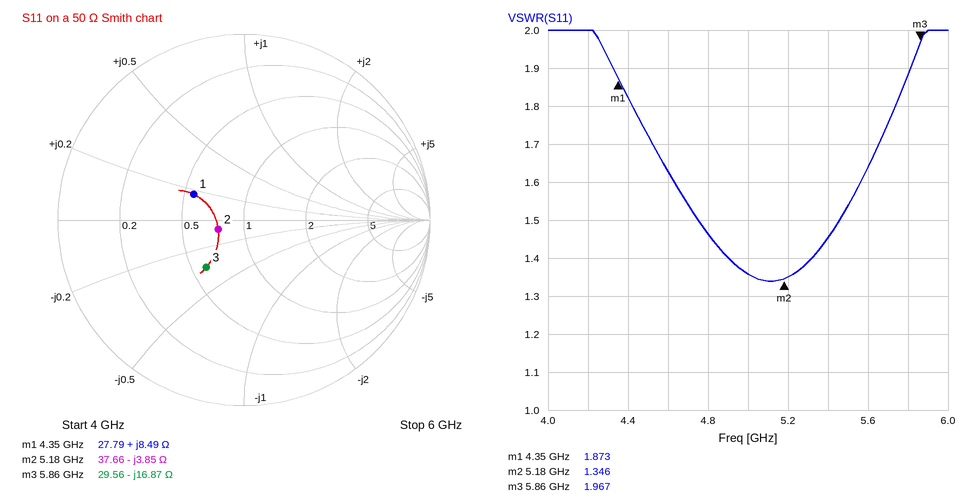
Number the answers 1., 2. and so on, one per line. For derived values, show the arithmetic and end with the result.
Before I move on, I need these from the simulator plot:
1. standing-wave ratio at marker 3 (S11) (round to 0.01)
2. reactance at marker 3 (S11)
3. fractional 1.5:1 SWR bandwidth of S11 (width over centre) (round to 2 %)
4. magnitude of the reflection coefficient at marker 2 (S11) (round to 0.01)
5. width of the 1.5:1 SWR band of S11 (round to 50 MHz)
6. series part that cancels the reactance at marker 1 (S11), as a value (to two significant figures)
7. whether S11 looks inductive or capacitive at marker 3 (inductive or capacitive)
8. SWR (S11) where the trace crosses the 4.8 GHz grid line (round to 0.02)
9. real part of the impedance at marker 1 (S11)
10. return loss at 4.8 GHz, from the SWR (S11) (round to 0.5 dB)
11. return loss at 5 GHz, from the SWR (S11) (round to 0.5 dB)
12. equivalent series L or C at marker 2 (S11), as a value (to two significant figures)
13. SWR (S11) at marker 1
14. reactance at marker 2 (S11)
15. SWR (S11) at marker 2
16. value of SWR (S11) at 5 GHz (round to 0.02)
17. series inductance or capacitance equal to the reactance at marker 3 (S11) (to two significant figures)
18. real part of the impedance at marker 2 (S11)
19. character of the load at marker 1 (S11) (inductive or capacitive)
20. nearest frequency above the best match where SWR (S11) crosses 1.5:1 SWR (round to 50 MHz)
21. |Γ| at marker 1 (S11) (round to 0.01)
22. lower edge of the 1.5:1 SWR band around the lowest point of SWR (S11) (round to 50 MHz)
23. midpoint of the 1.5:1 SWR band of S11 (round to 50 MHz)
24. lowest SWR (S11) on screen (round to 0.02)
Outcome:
1. 1.97
2. -16.87 Ω
3. 700 MHz / 5.1 GHz ≈ 14 %
4. 0.15
5. 5.45 GHz − 4.75 GHz = 700 MHz
6. C = 1/(2π × 4.35 GHz × 8.49 Ω) ≈ 4.3 pF
7. capacitive
8. 1.46
9. 27.79 Ω
10. −20 log10((1.46 − 1)/(1.46 + 1)) ≈ 14.6 dB, so 14.5 dB to the nearest 0.5 dB
11. −20 log10((1.36 − 1)/(1.36 + 1)) ≈ 16.3 dB, so 16.5 dB to the nearest 0.5 dB
12. C = 1/(2π × 5.18 GHz × 3.85 Ω) ≈ 8.0 pF
13. 1.873
14. -3.85 Ω
15. 1.346
16. 1.36
17. C = 1/(2π × 5.86 GHz × 16.87 Ω) ≈ 1.6 pF
18. 37.66 Ω
19. inductive
20. 5.45 GHz
21. 0.30
22. 4.75 GHz
23. 5.10 GHz
24. 1.34
